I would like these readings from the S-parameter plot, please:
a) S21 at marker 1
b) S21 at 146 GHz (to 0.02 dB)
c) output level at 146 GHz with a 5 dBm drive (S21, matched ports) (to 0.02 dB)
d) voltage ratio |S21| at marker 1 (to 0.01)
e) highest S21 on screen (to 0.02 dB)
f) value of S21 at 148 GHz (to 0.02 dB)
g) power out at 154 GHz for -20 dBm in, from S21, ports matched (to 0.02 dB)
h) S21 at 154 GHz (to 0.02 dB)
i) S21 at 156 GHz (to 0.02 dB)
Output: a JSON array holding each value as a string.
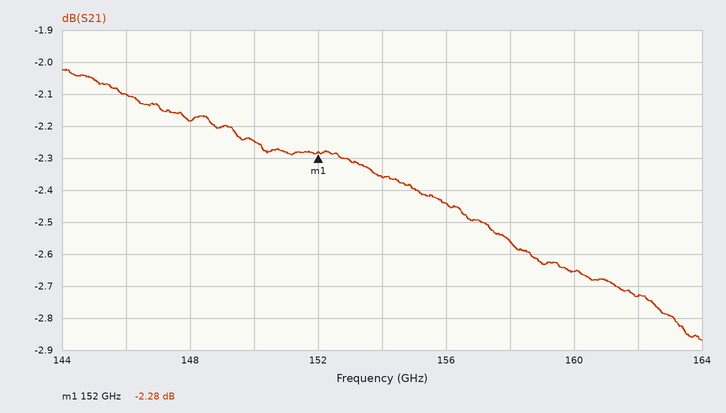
["-2.28 dB", "-2.10 dB", "2.90 dBm", "0.77", "-2.02 dB", "-2.18 dB", "-22.36 dBm", "-2.36 dB", "-2.44 dB"]
